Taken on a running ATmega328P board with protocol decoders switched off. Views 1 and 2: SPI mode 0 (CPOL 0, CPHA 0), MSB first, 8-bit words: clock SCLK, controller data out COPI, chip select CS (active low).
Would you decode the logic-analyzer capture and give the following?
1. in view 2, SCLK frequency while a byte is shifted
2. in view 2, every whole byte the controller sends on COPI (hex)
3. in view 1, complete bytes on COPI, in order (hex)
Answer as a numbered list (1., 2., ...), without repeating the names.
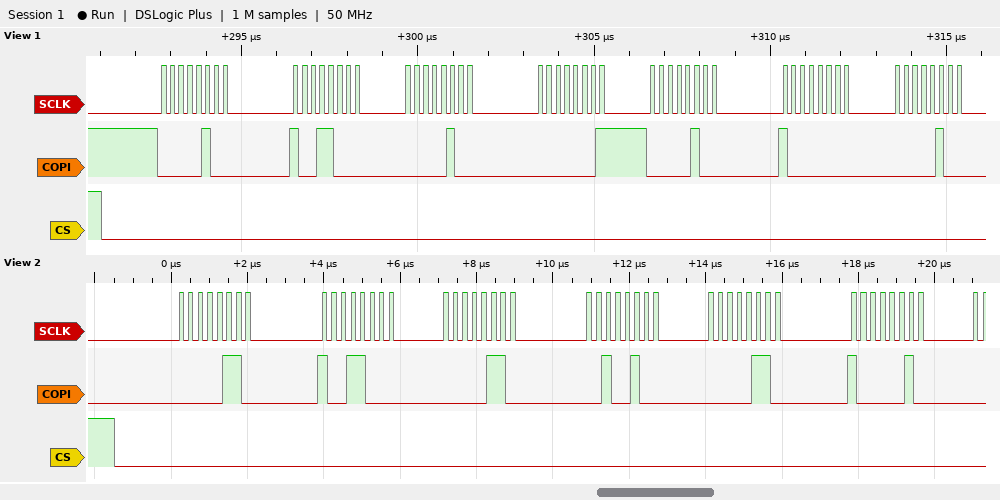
1. 4 MHz
2. 06 98 06 24 06 82
3. 04 98 04 01 04 80 04
